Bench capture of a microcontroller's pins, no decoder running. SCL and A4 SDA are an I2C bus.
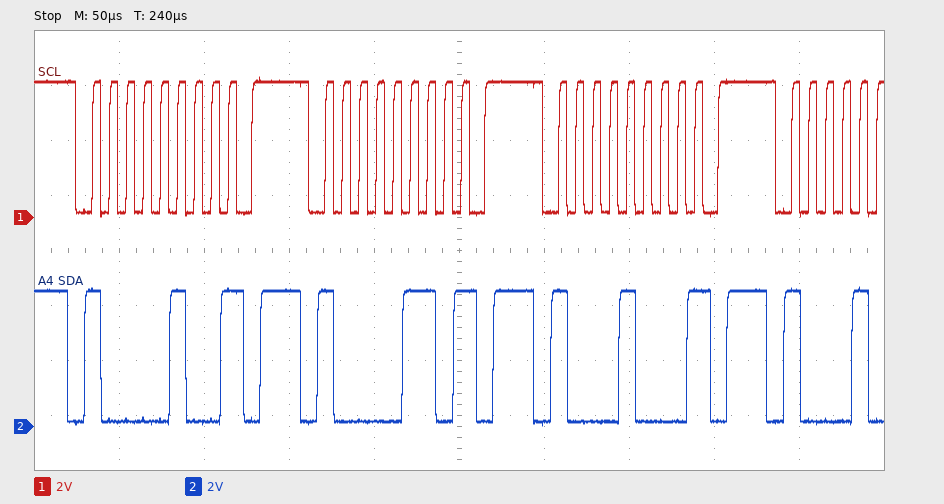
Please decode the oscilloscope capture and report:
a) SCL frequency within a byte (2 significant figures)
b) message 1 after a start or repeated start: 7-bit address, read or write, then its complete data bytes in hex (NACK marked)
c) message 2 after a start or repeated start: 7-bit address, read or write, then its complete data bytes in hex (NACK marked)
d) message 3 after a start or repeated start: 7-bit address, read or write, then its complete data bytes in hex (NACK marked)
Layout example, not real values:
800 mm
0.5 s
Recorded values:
100 kHz
0x42 write NACK
0x43 write NACK
0x44 write NACK
